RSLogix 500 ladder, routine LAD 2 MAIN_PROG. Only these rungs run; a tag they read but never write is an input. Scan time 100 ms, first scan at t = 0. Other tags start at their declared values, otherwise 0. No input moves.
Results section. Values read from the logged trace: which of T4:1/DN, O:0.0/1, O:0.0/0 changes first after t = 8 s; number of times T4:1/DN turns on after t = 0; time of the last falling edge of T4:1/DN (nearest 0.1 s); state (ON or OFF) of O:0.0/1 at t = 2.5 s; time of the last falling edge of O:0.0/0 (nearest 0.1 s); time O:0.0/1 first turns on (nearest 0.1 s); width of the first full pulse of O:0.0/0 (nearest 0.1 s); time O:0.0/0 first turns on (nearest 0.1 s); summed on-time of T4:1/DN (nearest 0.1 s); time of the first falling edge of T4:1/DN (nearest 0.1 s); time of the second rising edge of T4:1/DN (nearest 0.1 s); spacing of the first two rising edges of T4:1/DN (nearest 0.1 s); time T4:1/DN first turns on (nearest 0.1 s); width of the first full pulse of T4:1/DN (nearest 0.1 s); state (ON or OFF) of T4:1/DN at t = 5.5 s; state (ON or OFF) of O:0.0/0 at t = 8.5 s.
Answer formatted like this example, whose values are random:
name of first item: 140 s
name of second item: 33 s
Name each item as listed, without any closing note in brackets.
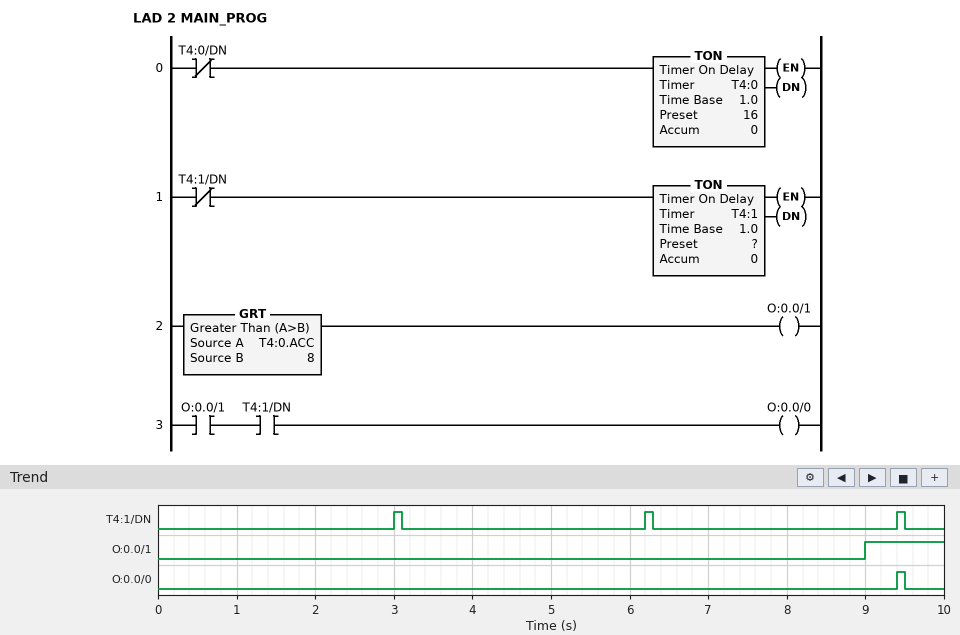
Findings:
which of T4:1/DN, O:0.0/1, O:0.0/0 changes first after t = 8 s: O:0.0/1
number of times T4:1/DN turns on after t = 0: 3
time of the last falling edge of T4:1/DN: 9.5 s
state (ON or OFF) of O:0.0/1 at t = 2.5 s: OFF
time of the last falling edge of O:0.0/0: 9.5 s
time O:0.0/1 first turns on: 9.0 s
width of the first full pulse of O:0.0/0: 0.1 s
time O:0.0/0 first turns on: 9.4 s
summed on-time of T4:1/DN: 0.3 s
time of the first falling edge of T4:1/DN: 3.1 s
time of the second rising edge of T4:1/DN: 6.2 s
spacing of the first two rising edges of T4:1/DN: 3.2 s
time T4:1/DN first turns on: 3.0 s
width of the first full pulse of T4:1/DN: 0.1 s
state (ON or OFF) of T4:1/DN at t = 5.5 s: OFF
state (ON or OFF) of O:0.0/0 at t = 8.5 s: OFF
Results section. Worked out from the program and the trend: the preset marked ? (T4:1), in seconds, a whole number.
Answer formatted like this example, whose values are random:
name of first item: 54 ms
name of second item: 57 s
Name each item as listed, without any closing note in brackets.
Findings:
the preset marked ? (T4:1), in seconds, a whole number: 3 s
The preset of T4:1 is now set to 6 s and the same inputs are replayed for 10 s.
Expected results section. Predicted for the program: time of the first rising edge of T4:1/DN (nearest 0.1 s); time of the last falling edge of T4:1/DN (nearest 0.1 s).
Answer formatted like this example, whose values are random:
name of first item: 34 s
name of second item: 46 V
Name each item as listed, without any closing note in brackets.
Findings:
time of the first rising edge of T4:1/DN: 6.0 s
time of the last falling edge of T4:1/DN: 6.1 s
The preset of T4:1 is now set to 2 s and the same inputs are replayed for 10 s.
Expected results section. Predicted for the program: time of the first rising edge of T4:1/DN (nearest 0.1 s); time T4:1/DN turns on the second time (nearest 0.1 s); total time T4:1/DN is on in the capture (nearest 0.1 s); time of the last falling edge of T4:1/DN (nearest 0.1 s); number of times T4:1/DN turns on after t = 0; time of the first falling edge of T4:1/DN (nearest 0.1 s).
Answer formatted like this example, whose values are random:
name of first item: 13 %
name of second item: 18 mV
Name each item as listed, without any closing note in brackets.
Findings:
time of the first rising edge of T4:1/DN: 2.0 s
time T4:1/DN turns on the second time: 4.2 s
total time T4:1/DN is on in the capture: 0.4 s
time of the last falling edge of T4:1/DN: 8.7 s
number of times T4:1/DN turns on after t = 0: 4
time of the first falling edge of T4:1/DN: 2.1 s
